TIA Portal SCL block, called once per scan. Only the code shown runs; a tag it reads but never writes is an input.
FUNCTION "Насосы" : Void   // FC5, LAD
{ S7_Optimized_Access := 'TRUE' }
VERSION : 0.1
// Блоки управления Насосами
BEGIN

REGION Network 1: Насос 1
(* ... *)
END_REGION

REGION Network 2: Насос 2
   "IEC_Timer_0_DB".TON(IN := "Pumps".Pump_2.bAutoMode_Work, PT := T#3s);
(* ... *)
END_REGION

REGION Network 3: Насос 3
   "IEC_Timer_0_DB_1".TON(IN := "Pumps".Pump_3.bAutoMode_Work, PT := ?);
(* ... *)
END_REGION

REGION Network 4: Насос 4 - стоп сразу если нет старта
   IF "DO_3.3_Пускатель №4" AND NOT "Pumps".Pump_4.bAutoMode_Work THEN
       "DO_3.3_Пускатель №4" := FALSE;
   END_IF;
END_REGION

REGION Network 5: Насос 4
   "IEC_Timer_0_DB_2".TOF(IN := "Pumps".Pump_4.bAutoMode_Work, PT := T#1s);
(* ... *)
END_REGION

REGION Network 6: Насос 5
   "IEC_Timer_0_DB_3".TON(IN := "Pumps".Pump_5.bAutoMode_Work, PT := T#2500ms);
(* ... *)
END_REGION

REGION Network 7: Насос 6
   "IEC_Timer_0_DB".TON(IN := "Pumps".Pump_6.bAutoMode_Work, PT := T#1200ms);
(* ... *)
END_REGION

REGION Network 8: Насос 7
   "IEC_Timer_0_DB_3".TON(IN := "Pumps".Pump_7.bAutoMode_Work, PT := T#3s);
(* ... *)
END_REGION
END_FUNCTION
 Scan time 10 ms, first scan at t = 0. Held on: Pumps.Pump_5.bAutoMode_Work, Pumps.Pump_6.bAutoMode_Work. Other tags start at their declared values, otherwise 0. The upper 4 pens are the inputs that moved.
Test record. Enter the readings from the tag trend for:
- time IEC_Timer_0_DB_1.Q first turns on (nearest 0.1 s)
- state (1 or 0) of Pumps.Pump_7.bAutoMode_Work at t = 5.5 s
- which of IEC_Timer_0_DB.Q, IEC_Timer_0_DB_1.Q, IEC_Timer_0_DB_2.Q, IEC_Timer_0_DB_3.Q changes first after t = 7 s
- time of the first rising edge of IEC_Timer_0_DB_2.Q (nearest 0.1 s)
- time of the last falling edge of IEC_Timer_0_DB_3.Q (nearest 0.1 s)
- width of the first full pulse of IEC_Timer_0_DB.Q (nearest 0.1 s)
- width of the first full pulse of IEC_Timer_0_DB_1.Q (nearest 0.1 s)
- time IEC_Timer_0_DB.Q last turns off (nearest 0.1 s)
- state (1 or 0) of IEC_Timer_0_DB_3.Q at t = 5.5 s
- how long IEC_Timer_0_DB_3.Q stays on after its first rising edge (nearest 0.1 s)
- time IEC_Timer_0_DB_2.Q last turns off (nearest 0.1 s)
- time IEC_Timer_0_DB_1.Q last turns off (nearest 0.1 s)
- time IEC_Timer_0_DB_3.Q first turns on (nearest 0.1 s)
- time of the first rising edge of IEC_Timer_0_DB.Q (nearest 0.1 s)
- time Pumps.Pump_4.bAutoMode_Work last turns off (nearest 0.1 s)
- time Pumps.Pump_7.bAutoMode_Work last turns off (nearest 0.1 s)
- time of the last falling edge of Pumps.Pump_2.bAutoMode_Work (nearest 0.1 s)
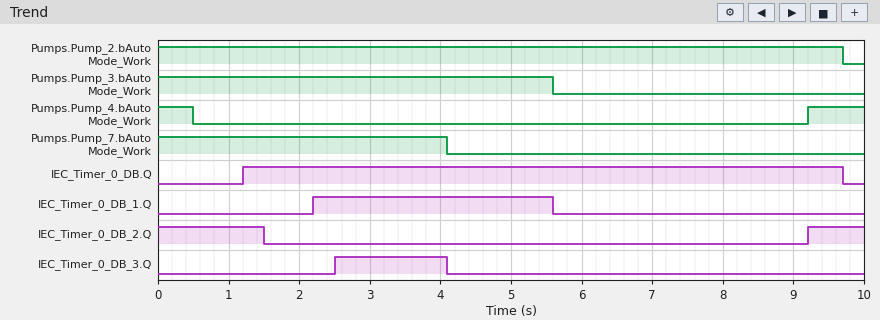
2.2 s
0
IEC_Timer_0_DB_2.Q
9.2 s
4.1 s
8.5 s
3.4 s
9.7 s
0
1.6 s
1.5 s
5.6 s
2.5 s
1.2 s
0.5 s
4.1 s
9.7 s
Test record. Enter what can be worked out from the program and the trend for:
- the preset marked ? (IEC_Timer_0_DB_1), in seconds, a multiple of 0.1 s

2.2 s
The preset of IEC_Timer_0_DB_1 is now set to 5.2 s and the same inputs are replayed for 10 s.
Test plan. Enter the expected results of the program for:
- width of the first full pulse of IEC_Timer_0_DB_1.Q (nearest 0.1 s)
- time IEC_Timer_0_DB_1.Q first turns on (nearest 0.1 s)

0.4 s
5.2 s
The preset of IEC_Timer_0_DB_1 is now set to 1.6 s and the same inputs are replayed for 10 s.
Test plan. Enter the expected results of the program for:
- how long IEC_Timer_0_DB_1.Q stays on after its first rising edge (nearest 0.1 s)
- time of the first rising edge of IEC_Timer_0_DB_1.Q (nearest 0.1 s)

4.0 s
1.6 s
